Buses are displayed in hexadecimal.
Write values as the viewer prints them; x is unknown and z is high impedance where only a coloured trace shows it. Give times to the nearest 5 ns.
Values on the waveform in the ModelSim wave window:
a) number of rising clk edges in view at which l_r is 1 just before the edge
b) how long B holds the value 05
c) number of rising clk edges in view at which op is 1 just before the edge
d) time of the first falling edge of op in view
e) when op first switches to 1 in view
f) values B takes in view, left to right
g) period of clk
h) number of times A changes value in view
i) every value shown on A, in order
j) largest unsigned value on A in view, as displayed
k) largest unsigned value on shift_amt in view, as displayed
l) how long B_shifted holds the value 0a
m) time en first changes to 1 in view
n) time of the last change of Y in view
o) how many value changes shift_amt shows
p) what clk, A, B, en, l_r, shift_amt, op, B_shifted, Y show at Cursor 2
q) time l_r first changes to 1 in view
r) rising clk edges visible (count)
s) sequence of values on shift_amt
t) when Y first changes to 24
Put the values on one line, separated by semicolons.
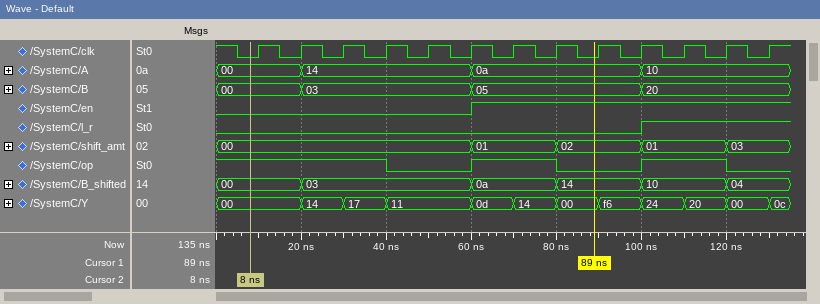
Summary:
3; 40 ns; 8; 40 ns; 60 ns; 00, 03, 05, 20; 10 ns; 3; 00, 14, 0a, 10; 14; 03; 20 ns; 60 ns; 130 ns; 4; clk=0, A=00, B=00, en=0, l_r=0, shift_amt=00, op=1, B_shifted=00, Y=00; 100 ns; 13; 00, 01, 02, 01, 03; 100 ns
